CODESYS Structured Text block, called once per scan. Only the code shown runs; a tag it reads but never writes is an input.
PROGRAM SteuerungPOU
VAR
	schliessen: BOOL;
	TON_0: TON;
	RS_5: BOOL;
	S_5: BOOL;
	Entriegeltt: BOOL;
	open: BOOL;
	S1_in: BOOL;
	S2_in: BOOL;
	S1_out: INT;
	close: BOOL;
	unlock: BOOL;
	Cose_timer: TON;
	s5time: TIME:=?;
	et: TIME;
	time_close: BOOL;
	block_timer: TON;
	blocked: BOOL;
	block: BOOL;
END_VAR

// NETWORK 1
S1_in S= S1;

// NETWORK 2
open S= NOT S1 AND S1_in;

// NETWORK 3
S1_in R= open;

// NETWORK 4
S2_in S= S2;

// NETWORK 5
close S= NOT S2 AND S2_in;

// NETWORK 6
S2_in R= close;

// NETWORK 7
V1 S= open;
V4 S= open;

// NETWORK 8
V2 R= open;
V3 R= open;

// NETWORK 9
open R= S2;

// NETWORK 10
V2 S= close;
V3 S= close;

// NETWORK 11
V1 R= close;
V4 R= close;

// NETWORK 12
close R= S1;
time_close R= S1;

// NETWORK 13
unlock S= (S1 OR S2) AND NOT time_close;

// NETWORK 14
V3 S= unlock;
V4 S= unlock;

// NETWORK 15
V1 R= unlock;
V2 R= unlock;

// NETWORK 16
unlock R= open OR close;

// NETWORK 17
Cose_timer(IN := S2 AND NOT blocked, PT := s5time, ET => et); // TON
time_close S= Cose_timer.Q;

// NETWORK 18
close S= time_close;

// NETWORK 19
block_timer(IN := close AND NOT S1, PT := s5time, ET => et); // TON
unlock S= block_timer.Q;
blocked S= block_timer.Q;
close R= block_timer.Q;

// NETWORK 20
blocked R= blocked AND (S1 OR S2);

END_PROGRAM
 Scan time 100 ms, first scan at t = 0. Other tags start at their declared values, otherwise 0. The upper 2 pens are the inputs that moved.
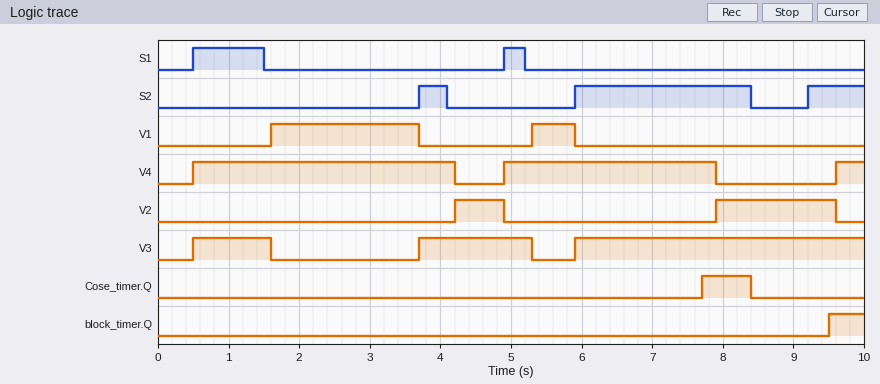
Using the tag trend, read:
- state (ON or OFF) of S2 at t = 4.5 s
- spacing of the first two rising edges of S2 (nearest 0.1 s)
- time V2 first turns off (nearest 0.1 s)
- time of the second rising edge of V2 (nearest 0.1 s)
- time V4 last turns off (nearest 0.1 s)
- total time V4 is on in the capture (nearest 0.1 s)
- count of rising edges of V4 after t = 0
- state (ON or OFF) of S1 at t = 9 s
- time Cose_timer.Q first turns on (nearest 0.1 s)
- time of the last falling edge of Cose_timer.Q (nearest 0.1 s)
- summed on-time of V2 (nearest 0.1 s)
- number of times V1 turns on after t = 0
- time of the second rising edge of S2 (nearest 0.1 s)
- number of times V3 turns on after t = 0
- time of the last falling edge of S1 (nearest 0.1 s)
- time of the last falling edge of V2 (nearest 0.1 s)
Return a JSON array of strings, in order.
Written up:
["OFF", "2.2 s", "4.9 s", "7.9 s", "7.9 s", "7.1 s", "3", "OFF", "7.7 s", "8.4 s", "2.4 s", "2", "5.9 s", "3", "5.2 s", "9.6 s"]
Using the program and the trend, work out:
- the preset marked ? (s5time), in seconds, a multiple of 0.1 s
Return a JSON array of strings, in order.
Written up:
["1.8 s"]
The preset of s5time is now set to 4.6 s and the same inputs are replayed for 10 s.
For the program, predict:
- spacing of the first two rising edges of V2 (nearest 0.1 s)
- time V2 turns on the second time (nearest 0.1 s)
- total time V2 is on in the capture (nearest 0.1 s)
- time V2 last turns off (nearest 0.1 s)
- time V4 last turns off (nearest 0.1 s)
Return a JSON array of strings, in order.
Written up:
["4.3 s", "8.5 s", "1.4 s", "9.2 s", "8.5 s"]
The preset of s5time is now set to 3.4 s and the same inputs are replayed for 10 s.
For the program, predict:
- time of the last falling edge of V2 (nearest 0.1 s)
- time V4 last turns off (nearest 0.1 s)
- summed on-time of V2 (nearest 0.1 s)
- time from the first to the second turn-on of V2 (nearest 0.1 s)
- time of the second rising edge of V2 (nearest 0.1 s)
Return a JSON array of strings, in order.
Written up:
["9.2 s", "8.5 s", "1.4 s", "4.3 s", "8.5 s"]
